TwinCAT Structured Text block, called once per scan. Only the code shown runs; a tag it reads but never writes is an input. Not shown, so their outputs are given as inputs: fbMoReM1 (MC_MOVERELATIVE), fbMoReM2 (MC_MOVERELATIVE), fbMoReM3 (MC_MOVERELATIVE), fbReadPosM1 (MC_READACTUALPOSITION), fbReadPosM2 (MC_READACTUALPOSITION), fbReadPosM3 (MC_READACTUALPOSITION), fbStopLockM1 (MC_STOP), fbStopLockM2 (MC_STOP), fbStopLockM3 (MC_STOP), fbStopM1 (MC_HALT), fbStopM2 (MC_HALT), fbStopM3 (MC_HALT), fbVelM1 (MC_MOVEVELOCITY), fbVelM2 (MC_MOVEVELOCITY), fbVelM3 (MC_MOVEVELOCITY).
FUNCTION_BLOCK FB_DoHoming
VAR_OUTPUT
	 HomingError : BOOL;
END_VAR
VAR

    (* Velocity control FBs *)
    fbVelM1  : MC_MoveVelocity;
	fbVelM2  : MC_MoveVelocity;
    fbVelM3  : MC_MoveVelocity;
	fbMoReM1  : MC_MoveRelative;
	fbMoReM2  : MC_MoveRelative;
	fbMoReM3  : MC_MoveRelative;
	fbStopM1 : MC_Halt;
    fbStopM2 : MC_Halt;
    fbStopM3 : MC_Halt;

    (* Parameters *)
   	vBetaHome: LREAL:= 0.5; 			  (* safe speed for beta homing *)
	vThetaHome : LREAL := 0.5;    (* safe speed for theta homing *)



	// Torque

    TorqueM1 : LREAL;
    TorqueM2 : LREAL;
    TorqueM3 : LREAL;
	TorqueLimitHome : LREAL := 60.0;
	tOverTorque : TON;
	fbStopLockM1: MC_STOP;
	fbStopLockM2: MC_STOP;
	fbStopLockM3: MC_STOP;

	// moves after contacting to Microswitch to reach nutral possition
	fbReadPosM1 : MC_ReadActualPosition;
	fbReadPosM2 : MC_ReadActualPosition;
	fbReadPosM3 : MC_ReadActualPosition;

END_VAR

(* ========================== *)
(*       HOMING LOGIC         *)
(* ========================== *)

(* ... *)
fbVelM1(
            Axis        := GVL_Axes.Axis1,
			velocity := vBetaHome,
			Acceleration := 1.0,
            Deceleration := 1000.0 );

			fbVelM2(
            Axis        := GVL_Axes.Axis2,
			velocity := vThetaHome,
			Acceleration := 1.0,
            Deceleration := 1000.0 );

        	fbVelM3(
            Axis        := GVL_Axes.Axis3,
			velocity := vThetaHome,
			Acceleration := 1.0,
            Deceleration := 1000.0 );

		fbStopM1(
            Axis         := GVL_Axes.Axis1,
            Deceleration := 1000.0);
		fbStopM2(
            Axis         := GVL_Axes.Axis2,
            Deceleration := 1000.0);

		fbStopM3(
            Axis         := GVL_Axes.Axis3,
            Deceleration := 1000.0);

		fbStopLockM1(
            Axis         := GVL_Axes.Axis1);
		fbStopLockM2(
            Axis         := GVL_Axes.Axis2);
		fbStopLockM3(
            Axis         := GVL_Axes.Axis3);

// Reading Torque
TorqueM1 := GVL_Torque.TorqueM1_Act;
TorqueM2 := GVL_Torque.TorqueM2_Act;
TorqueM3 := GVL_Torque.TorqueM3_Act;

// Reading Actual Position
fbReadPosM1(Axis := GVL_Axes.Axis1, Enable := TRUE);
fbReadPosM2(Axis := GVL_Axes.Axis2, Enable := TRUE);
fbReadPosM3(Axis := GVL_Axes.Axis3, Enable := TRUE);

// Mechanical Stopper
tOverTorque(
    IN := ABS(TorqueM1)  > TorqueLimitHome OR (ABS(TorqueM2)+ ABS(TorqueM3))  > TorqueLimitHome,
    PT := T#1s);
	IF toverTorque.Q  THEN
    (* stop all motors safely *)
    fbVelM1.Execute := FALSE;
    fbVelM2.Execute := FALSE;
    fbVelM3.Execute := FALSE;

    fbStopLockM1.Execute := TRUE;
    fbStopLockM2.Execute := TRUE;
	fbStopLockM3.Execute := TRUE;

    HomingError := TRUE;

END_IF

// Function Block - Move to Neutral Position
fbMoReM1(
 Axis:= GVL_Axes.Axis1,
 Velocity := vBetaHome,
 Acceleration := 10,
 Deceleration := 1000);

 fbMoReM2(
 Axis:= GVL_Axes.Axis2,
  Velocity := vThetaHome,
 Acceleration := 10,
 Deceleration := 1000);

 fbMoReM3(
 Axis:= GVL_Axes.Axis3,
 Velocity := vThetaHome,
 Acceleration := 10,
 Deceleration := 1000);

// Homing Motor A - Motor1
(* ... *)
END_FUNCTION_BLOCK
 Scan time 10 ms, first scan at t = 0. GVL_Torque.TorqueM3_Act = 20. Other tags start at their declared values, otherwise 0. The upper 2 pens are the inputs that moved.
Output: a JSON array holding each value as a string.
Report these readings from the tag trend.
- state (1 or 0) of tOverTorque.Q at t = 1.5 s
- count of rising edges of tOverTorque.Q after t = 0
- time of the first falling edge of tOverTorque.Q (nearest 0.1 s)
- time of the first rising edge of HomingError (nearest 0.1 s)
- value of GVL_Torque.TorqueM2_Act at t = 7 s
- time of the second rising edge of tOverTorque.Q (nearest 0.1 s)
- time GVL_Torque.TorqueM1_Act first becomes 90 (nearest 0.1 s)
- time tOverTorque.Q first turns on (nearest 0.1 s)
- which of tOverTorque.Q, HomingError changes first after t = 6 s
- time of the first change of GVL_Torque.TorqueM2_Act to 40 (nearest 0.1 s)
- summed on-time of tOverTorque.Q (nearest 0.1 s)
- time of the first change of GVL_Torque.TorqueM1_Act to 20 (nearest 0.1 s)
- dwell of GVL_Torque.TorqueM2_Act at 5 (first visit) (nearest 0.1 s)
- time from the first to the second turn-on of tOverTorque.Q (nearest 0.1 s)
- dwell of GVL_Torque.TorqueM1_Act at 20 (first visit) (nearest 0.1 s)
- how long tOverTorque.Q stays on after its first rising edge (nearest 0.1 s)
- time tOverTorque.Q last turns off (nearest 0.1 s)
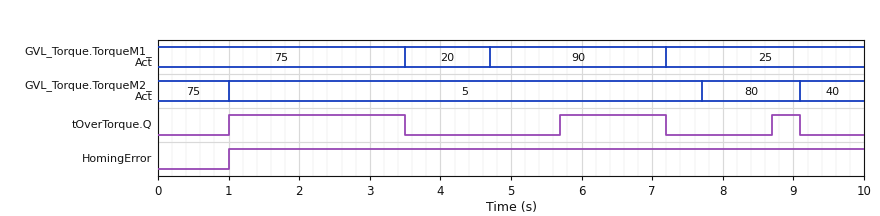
["1", "3", "3.5 s", "1.0 s", "5", "5.7 s", "4.7 s", "1.0 s", "tOverTorque.Q", "9.1 s", "4.4 s", "3.5 s", "6.7 s", "4.7 s", "1.2 s", "2.5 s", "9.1 s"]
